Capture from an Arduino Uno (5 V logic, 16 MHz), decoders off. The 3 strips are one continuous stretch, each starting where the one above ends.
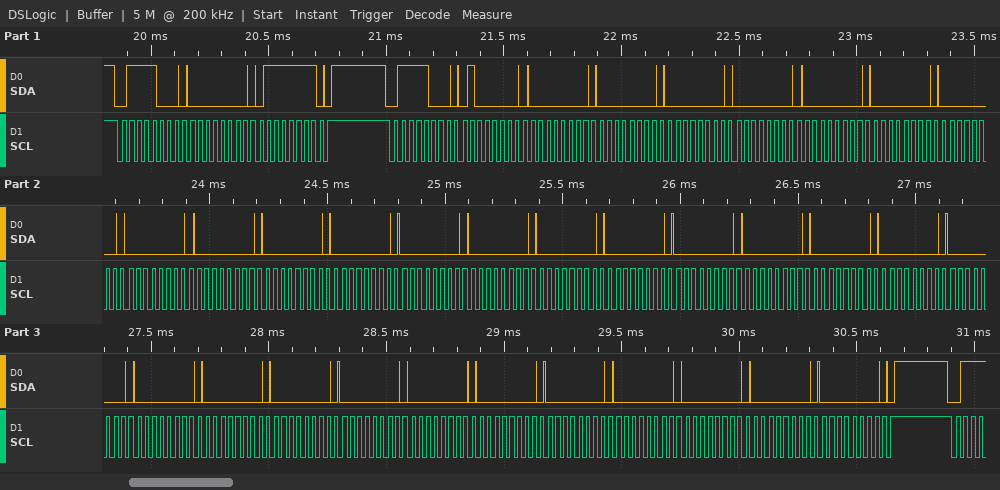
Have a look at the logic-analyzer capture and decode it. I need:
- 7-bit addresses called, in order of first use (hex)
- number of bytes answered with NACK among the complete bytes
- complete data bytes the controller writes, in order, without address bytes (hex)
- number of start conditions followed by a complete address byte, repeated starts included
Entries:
0x3C
0
00 7F 40 00 00 00 00 00 00 00 00 00 00 00 00 00 00 00 00 00 00 00 00 00 00 00 00 00 00 00 00 00 00 00
2
